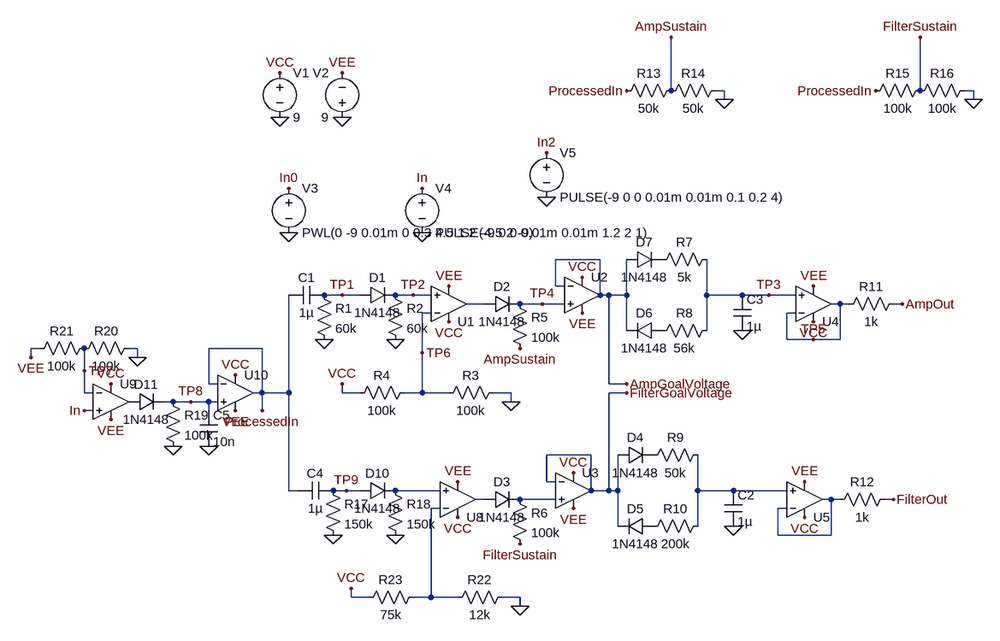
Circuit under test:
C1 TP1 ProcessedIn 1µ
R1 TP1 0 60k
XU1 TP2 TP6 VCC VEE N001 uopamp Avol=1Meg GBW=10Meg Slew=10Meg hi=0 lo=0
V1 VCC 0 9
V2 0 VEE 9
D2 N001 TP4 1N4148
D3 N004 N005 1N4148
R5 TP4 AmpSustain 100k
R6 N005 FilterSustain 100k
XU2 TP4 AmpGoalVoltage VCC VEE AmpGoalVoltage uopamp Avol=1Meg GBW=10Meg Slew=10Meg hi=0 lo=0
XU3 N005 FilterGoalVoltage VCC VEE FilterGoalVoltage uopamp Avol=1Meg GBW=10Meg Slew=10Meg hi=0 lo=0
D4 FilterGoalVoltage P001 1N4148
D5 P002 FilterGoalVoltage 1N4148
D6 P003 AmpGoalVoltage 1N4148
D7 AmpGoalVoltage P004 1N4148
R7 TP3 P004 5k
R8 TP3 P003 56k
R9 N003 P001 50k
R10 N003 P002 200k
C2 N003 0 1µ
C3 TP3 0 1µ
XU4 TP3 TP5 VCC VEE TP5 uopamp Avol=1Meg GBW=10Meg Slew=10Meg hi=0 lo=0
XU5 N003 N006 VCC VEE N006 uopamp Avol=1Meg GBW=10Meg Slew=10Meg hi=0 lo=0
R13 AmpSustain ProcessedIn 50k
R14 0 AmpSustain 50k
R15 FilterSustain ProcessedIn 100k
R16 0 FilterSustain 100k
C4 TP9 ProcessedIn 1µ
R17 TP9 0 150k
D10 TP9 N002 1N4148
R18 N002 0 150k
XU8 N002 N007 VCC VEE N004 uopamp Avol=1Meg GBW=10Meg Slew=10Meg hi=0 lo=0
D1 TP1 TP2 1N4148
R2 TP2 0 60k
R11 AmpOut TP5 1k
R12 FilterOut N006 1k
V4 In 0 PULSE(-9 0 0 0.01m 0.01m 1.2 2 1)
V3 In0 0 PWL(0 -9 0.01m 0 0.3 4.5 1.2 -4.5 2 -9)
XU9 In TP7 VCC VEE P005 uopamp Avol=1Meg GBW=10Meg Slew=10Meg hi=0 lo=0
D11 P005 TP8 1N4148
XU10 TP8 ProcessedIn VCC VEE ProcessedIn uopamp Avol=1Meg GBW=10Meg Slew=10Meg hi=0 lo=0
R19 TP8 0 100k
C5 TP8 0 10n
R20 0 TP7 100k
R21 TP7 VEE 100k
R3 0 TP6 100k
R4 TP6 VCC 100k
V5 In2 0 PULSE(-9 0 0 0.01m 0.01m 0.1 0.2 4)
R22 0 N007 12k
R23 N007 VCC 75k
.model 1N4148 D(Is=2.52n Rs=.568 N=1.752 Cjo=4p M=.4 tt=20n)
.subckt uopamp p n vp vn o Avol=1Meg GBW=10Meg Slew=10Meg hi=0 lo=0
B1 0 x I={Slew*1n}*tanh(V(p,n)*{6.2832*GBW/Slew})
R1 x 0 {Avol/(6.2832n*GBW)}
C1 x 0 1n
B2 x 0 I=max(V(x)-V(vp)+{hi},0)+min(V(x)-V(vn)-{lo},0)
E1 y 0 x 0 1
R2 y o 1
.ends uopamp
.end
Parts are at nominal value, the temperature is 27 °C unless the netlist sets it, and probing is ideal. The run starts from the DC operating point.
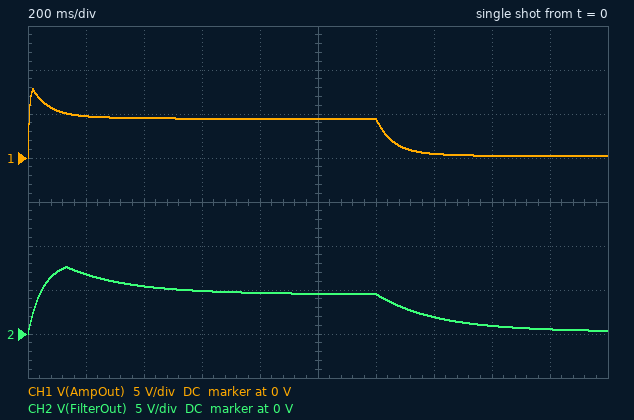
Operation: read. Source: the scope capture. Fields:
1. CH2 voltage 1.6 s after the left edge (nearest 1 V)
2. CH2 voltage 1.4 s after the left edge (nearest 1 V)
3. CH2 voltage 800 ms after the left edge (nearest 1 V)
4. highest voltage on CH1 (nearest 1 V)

1 V
2 V
5 V
8 V
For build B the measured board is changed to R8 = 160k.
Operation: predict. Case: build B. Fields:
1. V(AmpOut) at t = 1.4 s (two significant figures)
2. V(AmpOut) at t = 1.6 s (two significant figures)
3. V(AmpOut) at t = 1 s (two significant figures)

1.6 V
680 mV
4.5 V
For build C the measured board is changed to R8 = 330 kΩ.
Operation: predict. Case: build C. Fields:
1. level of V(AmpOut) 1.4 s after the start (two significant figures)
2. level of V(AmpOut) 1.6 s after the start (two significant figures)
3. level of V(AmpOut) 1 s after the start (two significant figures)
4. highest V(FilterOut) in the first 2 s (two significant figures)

2.7 V
1.6 V
4.7 V
7.6 V
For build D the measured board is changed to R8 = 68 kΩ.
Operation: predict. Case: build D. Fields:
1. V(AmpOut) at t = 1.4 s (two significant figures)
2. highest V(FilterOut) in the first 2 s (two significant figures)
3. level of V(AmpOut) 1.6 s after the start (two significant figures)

580 mV
7.6 V
280 mV
